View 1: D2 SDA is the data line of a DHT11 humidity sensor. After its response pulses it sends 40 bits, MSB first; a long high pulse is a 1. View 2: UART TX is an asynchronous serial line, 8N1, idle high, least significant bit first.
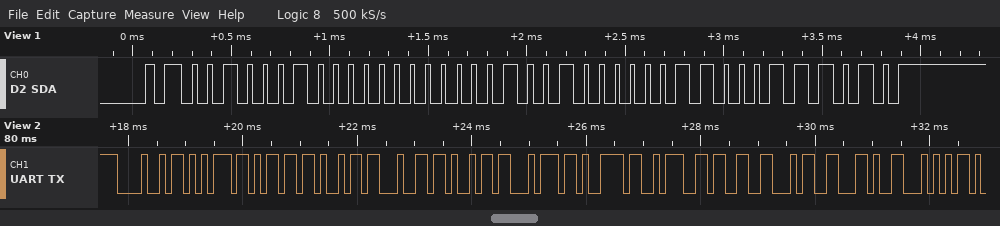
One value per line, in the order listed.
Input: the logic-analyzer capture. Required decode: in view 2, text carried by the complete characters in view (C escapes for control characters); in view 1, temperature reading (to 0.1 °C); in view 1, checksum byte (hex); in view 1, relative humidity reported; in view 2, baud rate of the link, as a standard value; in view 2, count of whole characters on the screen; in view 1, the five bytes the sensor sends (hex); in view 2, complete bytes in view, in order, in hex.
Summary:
"Humidity:34,T"
18.6 °C
0x3A
34 %
9600 baud
13
22 00 12 06 3A
48 75 6D 69 64 69 74 79 3A 33 34 2C 54
